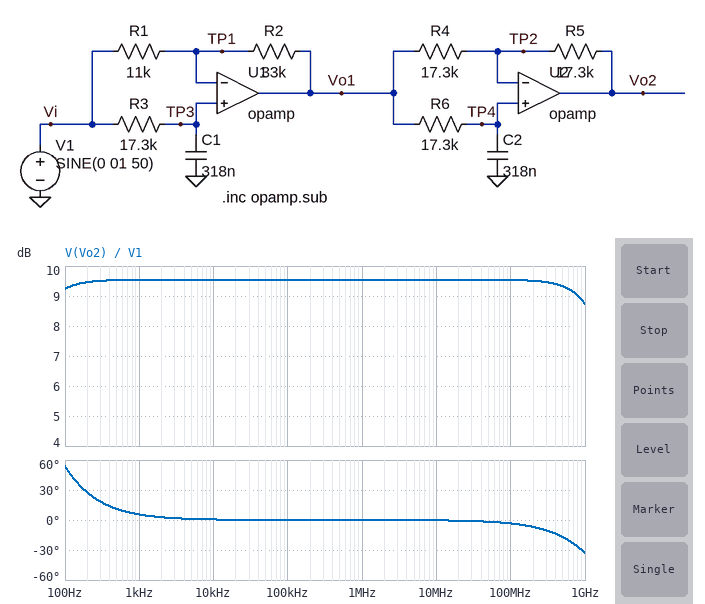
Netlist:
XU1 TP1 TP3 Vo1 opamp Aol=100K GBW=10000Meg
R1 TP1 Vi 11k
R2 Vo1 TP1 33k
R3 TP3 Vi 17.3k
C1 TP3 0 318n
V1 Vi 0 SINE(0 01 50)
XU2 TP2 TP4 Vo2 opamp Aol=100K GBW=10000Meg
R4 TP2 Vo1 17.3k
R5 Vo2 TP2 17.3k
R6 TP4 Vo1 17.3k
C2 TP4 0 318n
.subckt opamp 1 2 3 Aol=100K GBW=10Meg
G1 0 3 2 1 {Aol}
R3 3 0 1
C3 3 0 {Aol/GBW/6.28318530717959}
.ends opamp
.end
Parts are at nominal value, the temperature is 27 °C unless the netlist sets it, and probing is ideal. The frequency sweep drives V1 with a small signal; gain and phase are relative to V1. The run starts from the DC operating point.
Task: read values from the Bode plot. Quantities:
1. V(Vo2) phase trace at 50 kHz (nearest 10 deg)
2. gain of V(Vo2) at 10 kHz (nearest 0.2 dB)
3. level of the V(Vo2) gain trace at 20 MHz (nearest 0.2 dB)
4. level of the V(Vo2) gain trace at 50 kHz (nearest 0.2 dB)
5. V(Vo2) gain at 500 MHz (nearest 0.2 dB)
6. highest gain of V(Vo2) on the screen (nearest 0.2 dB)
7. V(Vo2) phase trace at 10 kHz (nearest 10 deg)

0 deg
9.6 dB
9.6 dB
9.6 dB
9.4 dB
9.6 dB
0 deg
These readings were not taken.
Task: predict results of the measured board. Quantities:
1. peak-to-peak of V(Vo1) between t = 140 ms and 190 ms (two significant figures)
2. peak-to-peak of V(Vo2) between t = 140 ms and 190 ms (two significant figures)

5.3 V
5.3 V
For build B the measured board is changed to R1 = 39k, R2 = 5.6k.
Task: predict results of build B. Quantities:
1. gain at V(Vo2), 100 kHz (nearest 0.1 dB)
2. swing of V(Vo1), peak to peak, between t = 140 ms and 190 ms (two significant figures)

-16.9 dB
1.0 V
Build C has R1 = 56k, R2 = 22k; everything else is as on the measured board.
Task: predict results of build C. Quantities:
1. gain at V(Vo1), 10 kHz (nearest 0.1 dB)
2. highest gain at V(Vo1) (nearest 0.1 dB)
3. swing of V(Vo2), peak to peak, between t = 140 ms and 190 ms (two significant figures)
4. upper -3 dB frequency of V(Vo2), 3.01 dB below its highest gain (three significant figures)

-8.1 dB
0 dB
1.2 V
34.8 Hz
